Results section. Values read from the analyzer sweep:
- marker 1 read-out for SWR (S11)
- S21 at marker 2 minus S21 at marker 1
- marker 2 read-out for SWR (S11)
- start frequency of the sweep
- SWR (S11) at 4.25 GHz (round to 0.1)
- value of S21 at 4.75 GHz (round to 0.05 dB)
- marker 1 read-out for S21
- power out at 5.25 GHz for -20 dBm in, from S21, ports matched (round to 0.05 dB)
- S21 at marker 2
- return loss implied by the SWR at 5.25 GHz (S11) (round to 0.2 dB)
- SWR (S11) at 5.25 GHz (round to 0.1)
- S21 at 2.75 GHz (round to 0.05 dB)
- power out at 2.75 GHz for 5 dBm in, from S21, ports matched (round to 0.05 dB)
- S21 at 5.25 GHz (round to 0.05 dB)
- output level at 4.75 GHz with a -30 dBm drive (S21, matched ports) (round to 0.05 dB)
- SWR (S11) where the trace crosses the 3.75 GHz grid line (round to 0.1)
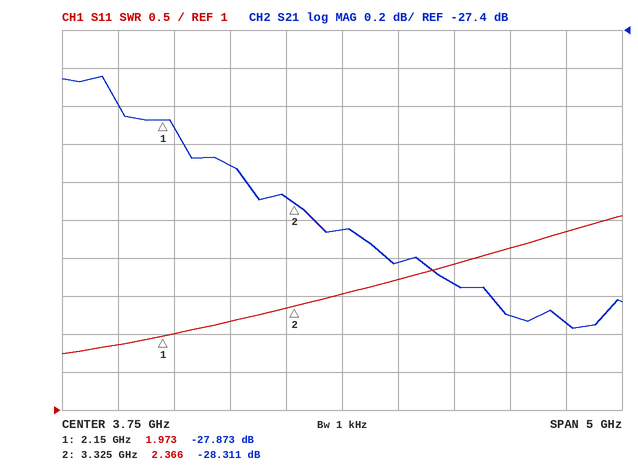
1.973
-0.438 dB
2.366
1.25 GHz
2.7
-28.75 dB
-27.873 dB
-48.90 dBm
-28.311 dB
5.8 dB
3.1
-28.10 dB
-23.10 dBm
-28.90 dB
-58.75 dBm
2.5
